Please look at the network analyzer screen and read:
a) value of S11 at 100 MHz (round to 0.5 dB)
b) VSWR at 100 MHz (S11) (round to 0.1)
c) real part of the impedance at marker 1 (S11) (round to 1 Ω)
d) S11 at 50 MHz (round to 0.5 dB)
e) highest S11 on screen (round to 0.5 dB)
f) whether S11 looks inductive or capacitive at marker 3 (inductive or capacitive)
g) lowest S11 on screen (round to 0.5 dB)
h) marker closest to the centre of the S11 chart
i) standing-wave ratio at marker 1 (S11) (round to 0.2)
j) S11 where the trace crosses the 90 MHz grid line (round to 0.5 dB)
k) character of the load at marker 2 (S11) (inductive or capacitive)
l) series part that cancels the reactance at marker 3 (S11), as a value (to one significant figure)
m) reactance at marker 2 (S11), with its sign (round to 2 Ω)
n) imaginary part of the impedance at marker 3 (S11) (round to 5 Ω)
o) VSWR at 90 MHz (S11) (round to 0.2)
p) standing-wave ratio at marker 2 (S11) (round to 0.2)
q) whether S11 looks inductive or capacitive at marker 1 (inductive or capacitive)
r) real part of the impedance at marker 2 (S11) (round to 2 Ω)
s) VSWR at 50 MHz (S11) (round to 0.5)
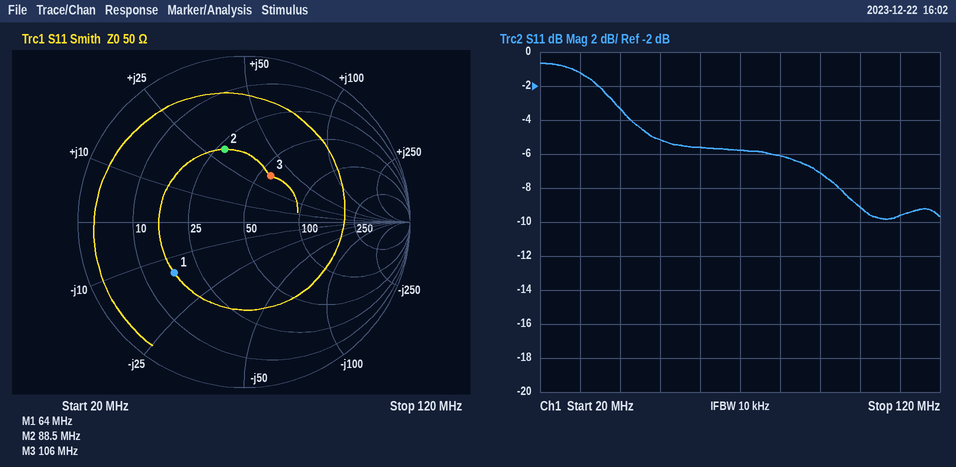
-9.0 dB
2.1
17 Ω
-5.0 dB
-0.5 dB
inductive
-10.0 dB
marker 3
3.2
-7.0 dB
inductive
40 pF
+30 Ω
+35 Ω
2.6
2.6
capacitive
28 Ω
3.5
